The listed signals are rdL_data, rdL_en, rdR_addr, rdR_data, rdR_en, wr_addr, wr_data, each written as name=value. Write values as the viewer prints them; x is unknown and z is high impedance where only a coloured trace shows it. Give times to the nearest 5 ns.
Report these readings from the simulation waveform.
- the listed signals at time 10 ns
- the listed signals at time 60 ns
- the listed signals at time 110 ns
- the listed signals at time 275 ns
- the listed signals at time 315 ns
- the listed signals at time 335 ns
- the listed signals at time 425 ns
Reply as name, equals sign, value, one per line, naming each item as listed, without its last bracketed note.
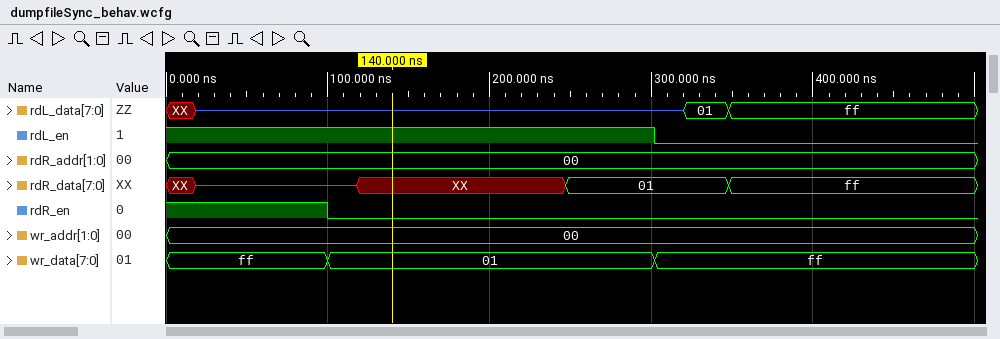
the listed signals at time 10 ns = rdL_data=XX, rdL_en=1, rdR_addr=00, rdR_data=XX, rdR_en=1, wr_addr=00, wr_data=ff
the listed signals at time 60 ns = rdL_data=z, rdL_en=1, rdR_addr=00, rdR_data=z, rdR_en=1, wr_addr=00, wr_data=ff
the listed signals at time 110 ns = rdL_data=z, rdL_en=1, rdR_addr=00, rdR_data=z, rdR_en=0, wr_addr=00, wr_data=01
the listed signals at time 275 ns = rdL_data=z, rdL_en=1, rdR_addr=00, rdR_data=01, rdR_en=0, wr_addr=00, wr_data=01
the listed signals at time 315 ns = rdL_data=z, rdL_en=0, rdR_addr=00, rdR_data=01, rdR_en=0, wr_addr=00, wr_data=ff
the listed signals at time 335 ns = rdL_data=01, rdL_en=0, rdR_addr=00, rdR_data=01, rdR_en=0, wr_addr=00, wr_data=ff
the listed signals at time 425 ns = rdL_data=ff, rdL_en=0, rdR_addr=00, rdR_data=ff, rdR_en=0, wr_addr=00, wr_data=ff
